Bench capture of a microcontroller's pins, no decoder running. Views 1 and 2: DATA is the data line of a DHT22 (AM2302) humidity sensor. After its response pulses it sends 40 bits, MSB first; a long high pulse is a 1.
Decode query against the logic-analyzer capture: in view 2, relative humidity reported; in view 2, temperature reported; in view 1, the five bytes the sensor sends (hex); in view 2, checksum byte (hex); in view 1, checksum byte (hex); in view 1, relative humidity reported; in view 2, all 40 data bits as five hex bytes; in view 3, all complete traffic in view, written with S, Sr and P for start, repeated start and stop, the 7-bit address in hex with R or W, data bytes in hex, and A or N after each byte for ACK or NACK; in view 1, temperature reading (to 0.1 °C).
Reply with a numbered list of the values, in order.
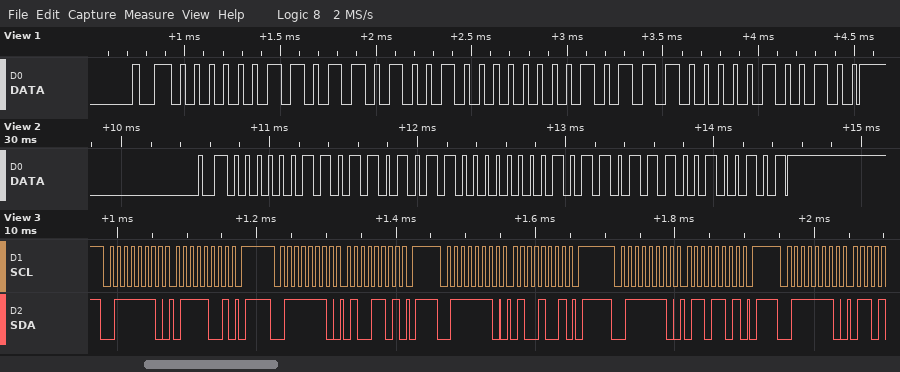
1. 87.5 %
2. 18.3 °C
3. 03 69 00 B8 24
4. 0x25
5. 0x24
6. 87.3 %
7. 03 6B 00 B7 25
8. S 3FW A 79 A P S 3FW A 4D A P S 3FW A 49 A P S 3FW A 6D A P S 3FW A
9. 18.4 °C
